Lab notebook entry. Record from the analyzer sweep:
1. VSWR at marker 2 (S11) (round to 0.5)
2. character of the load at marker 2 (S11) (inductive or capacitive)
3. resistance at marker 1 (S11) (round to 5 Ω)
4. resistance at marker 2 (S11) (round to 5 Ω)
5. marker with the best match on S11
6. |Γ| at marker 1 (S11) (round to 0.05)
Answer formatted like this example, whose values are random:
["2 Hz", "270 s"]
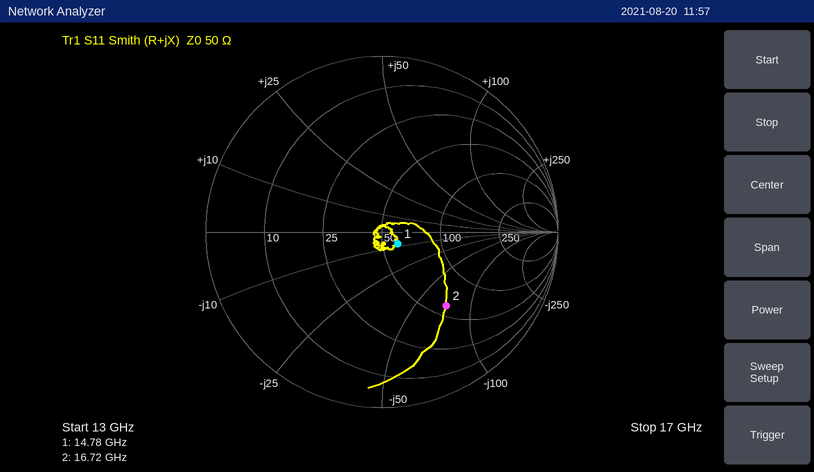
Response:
["3.5", "capacitive", "60 Ω", "60 Ω", "marker 1", "0.10"]
